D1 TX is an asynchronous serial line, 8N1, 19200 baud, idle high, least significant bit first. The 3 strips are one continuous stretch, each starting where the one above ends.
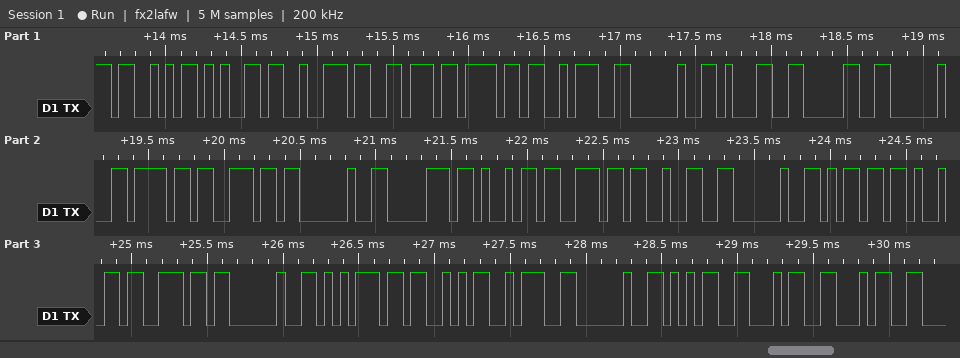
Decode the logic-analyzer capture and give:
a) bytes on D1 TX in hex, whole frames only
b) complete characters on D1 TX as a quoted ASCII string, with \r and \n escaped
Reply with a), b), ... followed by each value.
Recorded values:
a) 53 65 72 76 6F 3A 20 31 30 20 6F 6E 20 70 69 6E 32 20 6D 69 6E 20 75 53 3A 20 35 34 34
b) "Servo: 10 on pin2 min uS: 544"
